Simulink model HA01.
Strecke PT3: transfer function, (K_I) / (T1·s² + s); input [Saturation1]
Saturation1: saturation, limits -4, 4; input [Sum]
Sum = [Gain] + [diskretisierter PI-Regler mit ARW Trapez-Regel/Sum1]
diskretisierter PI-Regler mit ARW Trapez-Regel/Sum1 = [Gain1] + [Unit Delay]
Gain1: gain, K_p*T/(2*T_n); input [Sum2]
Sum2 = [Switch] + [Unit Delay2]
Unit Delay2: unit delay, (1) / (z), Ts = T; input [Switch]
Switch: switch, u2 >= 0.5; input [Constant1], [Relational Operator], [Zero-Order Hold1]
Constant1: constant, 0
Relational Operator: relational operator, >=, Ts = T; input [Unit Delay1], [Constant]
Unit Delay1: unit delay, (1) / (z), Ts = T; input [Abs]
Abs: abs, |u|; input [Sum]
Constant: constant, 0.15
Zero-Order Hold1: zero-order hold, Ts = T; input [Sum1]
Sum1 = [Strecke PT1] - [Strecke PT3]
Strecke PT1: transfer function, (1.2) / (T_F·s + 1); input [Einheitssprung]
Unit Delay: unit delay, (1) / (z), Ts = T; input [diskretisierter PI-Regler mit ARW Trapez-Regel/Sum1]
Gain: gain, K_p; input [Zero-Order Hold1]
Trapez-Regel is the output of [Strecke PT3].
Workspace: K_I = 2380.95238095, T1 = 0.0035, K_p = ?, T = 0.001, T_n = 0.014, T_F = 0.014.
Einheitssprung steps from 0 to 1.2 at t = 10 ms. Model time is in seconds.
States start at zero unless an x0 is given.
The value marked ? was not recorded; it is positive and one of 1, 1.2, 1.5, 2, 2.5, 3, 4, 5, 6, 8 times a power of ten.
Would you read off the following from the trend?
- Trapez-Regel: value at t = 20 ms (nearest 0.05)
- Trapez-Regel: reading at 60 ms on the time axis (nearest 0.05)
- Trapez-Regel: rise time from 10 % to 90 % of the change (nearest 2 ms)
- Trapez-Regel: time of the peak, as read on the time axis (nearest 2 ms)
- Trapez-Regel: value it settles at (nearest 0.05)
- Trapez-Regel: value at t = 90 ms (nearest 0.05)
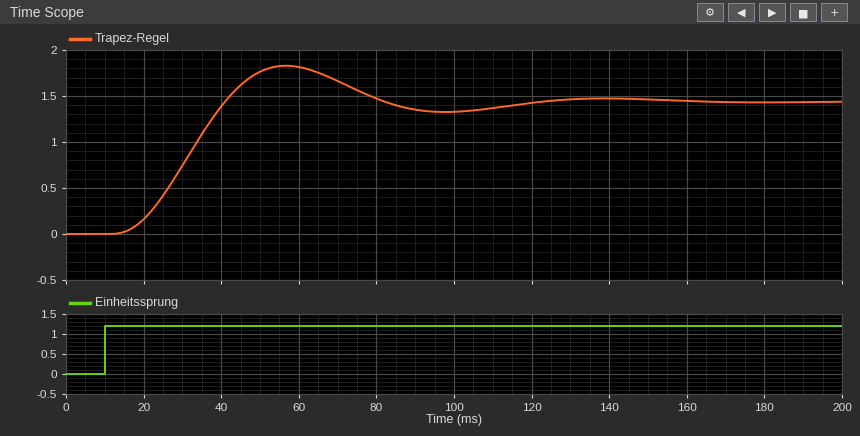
0.15
1.80
18 ms
56 ms
1.45
1.35
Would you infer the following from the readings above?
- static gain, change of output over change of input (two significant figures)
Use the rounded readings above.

1.2
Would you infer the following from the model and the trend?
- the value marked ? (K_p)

0.03
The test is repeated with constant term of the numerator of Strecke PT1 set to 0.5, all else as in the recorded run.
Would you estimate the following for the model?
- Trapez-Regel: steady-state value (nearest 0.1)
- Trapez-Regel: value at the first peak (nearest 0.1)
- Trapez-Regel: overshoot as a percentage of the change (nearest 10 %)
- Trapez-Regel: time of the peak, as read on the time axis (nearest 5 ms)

0.6
0.8
30 %
55 ms
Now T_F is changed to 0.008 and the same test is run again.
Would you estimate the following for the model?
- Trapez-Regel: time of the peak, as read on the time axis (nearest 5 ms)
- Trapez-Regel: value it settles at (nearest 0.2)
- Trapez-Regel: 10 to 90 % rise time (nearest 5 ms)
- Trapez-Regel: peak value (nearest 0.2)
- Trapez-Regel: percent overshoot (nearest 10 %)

50 ms
1.4
15 ms
2.0
40 %
